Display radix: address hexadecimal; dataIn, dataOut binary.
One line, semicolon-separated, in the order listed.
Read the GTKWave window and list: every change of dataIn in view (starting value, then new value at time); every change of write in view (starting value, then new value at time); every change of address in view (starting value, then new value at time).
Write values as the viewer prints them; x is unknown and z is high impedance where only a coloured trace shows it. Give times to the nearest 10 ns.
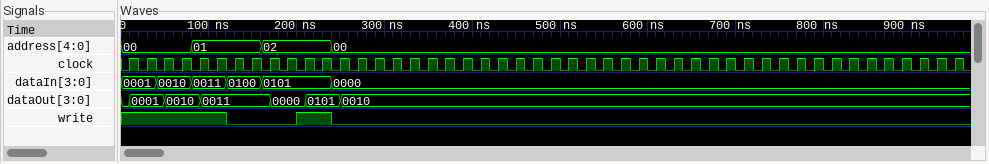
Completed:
0001, 0010 at 40 ns, 0011 at 80 ns, 0100 at 120 ns, 0101 at 160 ns, 0000 at 240 ns; 1, 0 at 120 ns, 1 at 200 ns, 0 at 240 ns; 00, 01 at 80 ns, 02 at 160 ns, 00 at 240 ns
